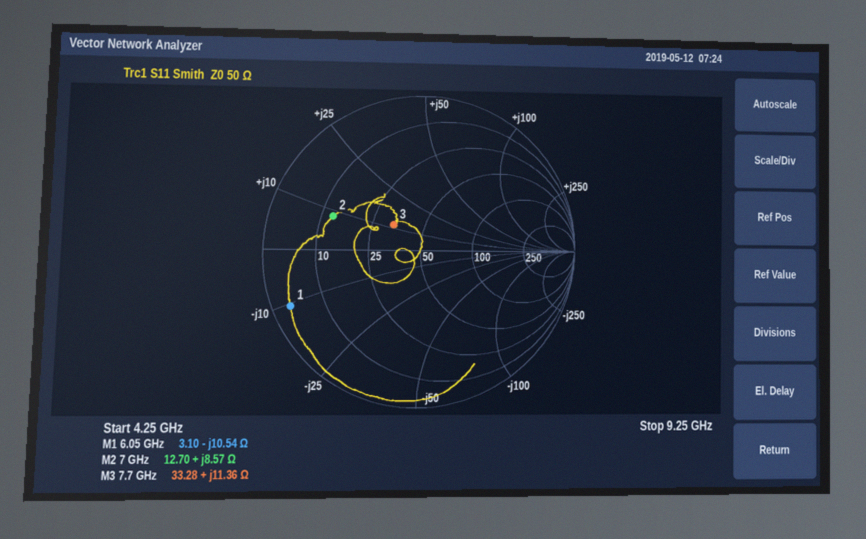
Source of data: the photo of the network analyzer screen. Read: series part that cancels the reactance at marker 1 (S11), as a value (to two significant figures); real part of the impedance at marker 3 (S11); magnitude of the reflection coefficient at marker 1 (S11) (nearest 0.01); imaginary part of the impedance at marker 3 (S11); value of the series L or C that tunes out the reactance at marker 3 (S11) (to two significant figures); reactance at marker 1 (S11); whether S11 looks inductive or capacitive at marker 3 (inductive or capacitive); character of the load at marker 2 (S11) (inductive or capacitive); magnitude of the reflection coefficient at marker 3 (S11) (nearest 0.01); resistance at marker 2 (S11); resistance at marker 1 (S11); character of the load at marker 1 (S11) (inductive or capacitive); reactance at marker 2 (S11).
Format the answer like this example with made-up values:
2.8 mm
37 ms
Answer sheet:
280 pH
33.28 Ω
0.89
+11.36 Ω
1.8 pF
-10.54 Ω
inductive
inductive
0.24
12.70 Ω
3.10 Ω
capacitive
+8.57 Ω
